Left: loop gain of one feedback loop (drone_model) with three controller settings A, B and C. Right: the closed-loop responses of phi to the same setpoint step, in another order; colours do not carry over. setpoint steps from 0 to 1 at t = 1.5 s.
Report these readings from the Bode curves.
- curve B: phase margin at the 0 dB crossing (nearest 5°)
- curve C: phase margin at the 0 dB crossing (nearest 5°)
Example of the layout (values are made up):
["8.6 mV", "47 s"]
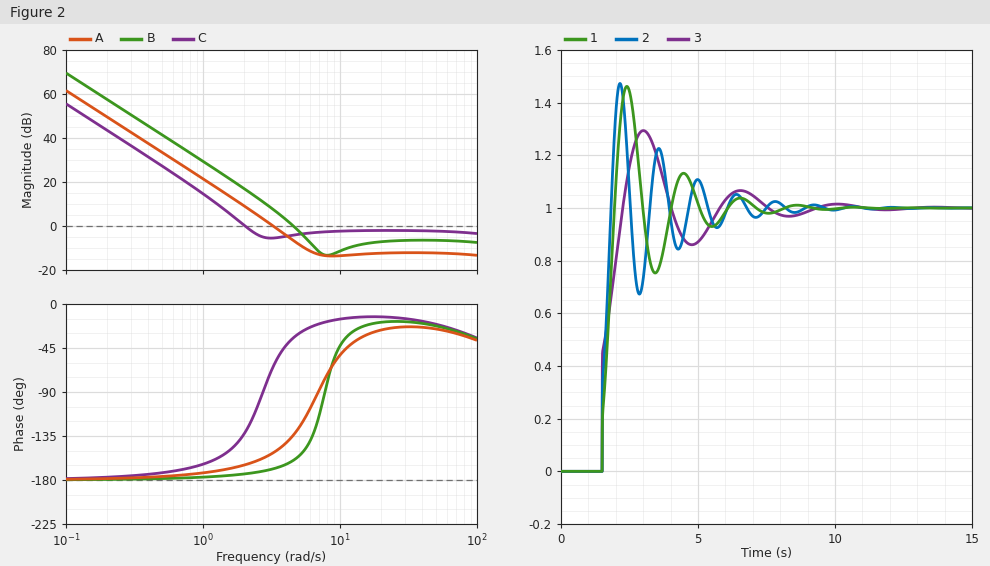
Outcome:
["20°", "50°"]
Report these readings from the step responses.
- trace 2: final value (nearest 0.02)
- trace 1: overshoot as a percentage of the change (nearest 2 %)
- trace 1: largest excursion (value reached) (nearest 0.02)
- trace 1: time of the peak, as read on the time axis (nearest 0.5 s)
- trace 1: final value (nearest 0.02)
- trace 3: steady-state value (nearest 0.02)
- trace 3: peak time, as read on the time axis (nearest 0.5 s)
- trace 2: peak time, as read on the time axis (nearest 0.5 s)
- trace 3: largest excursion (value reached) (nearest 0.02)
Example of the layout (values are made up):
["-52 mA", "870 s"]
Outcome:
["1.00", "46 %", "1.46", "2.5 s", "1.00", "1.00", "3.0 s", "2.0 s", "1.30"]
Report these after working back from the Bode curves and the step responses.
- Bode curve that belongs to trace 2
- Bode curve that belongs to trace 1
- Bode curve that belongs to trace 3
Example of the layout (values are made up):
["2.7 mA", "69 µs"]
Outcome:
["B", "A", "C"]
